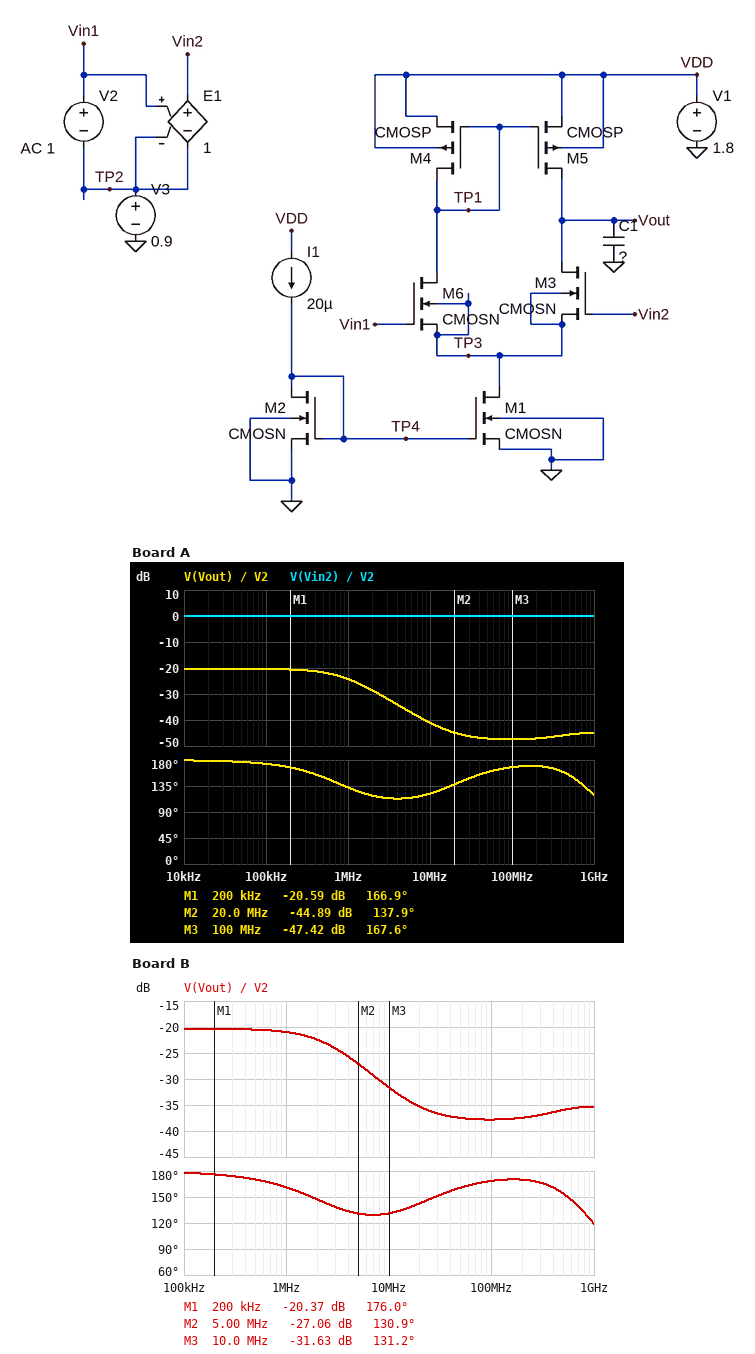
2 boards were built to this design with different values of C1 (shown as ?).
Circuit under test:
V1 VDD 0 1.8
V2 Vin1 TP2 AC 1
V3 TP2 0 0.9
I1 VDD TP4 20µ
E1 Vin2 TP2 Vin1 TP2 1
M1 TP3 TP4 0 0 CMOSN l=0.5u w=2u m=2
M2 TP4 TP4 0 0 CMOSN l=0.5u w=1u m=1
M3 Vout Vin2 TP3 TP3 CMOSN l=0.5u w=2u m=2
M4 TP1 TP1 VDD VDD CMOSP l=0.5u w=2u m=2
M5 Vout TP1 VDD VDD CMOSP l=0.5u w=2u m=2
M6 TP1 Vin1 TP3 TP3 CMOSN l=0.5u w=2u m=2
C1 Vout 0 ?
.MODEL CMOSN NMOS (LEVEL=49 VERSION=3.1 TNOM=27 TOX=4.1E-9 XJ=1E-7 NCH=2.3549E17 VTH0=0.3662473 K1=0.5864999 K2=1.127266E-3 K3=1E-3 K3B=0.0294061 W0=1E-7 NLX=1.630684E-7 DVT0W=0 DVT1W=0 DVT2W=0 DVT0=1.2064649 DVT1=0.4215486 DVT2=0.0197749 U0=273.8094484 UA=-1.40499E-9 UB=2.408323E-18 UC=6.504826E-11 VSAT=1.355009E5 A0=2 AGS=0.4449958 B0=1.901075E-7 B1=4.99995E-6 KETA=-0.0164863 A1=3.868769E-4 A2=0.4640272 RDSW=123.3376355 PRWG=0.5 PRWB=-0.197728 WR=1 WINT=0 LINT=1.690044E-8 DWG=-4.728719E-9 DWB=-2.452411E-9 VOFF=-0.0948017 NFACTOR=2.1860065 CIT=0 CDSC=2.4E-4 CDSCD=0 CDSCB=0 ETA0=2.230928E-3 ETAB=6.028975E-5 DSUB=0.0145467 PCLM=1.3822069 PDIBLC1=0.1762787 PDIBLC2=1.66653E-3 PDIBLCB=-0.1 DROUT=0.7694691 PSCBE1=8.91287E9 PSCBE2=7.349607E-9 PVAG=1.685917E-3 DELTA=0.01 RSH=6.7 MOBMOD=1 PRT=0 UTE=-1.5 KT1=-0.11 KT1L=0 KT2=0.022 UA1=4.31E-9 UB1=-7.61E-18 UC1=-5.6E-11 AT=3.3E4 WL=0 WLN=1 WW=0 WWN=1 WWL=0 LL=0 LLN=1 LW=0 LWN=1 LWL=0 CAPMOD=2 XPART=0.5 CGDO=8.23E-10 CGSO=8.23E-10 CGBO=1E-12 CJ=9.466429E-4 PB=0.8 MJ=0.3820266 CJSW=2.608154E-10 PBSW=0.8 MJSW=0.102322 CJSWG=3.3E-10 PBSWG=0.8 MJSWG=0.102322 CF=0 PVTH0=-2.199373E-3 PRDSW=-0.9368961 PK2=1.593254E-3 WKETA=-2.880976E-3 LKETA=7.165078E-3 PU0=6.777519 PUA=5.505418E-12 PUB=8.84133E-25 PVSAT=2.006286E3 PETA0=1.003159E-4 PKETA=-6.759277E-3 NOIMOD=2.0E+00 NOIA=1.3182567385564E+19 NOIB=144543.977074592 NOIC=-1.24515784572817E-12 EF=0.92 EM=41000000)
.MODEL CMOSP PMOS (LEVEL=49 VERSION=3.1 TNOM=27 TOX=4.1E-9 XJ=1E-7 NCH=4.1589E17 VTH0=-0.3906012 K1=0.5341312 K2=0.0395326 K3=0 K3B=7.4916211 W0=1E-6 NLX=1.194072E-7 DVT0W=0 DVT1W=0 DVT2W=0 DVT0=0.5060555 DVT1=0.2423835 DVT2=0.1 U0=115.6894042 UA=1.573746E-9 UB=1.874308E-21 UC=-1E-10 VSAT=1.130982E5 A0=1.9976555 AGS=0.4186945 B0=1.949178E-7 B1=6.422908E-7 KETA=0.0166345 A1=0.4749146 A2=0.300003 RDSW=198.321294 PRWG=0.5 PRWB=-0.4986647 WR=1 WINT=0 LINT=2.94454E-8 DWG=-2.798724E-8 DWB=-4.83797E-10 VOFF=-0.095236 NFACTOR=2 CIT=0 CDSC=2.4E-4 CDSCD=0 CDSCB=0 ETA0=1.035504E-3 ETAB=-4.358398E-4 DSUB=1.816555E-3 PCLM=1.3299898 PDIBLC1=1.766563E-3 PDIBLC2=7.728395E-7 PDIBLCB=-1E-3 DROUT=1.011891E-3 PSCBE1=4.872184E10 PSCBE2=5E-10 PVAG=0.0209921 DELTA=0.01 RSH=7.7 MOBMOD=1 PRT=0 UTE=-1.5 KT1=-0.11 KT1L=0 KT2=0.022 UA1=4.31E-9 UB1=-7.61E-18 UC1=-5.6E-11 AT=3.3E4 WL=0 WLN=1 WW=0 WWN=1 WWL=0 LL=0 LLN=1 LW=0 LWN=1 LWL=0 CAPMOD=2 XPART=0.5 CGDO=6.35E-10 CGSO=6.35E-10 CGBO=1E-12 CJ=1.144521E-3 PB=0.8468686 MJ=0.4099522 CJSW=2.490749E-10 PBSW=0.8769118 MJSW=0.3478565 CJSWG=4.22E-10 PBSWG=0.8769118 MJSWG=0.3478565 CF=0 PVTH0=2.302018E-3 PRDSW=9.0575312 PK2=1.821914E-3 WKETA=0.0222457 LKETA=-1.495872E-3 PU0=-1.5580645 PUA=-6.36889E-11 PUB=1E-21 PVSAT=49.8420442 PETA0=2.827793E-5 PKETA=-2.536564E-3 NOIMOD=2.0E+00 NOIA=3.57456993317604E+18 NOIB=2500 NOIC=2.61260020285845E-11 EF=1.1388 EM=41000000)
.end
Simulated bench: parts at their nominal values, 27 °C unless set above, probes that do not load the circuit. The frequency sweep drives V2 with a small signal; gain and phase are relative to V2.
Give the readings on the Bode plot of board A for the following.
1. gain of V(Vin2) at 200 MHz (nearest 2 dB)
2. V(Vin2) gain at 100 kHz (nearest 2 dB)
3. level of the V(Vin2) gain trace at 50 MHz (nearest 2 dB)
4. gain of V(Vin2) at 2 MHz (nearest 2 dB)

0 dB
0 dB
0 dB
0 dB
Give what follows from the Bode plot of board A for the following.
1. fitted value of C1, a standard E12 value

1.2 pF
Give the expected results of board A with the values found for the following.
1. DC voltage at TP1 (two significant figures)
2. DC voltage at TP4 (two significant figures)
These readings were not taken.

980 mV
720 mV
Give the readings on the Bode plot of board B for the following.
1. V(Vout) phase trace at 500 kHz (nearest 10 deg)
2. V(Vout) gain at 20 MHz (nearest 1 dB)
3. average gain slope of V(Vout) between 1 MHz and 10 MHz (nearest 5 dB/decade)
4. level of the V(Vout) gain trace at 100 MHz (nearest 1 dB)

170 deg
-35 dB
-10 dB/decade
-38 dB
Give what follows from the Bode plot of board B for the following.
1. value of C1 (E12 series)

390 fF
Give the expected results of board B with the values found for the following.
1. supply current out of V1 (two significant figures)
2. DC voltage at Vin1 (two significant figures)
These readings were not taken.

91 µA
900 mV
